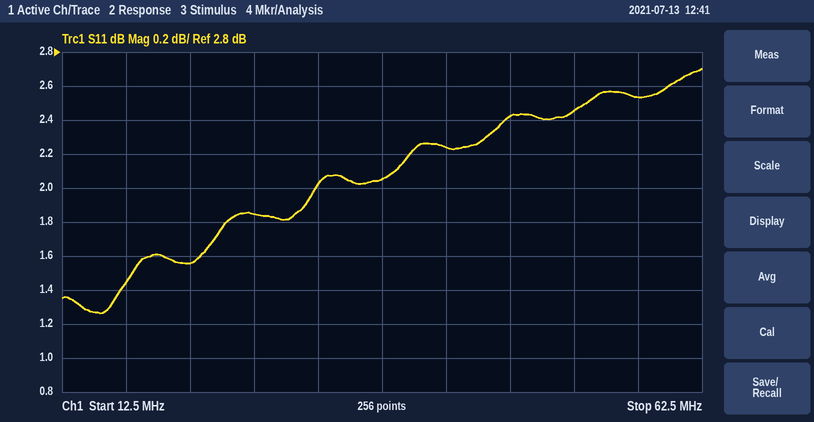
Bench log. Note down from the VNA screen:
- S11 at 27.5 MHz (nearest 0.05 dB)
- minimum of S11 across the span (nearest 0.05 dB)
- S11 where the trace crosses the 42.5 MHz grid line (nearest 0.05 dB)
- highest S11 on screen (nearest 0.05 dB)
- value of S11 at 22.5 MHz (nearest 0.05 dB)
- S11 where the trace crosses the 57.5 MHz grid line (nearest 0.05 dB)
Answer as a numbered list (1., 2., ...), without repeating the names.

1. 1.85 dB
2. 1.25 dB
3. 2.25 dB
4. 2.70 dB
5. 1.55 dB
6. 2.55 dB
